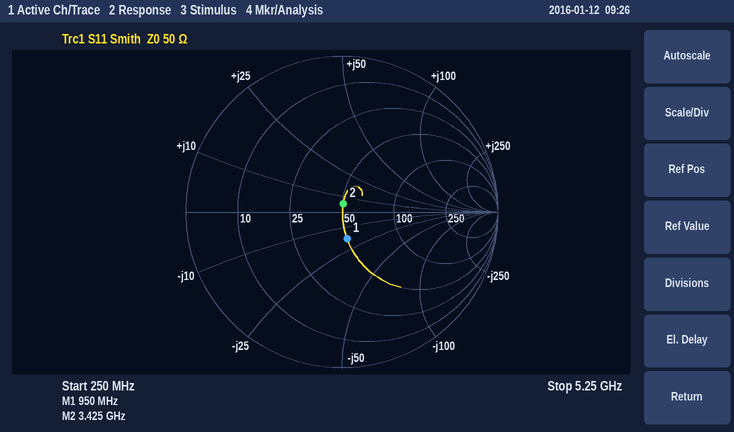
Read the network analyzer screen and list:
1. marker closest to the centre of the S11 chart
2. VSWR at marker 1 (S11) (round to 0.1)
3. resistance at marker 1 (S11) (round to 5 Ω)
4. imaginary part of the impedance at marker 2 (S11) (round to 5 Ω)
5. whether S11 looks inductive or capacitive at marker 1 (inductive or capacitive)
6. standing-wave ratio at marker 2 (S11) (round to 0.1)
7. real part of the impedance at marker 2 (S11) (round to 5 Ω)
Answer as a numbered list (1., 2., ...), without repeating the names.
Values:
1. marker 2
2. 1.4
3. 50 Ω
4. +5 Ω
5. capacitive
6. 1.1
7. 50 Ω
